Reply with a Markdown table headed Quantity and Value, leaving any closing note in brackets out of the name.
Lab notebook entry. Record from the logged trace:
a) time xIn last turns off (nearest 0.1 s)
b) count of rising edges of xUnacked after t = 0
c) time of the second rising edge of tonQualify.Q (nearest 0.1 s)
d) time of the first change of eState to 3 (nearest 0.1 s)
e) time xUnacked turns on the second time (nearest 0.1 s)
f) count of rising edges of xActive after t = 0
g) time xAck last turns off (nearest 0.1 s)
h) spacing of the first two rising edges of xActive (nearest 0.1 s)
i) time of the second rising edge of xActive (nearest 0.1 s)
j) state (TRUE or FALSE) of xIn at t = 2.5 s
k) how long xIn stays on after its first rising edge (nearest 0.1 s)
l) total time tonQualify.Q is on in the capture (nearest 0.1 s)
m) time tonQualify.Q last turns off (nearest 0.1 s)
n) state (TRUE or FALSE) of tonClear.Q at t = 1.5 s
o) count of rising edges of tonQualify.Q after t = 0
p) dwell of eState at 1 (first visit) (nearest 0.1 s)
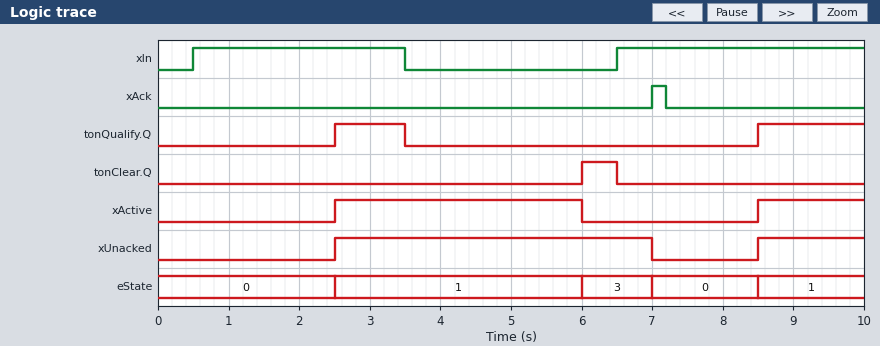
| Quantity | Value |
|---|---|
| time xIn last turns off | 3.5 s |
| count of rising edges of xUnacked after t = 0 | 2 |
| time of the second rising edge of tonQualify.Q | 8.5 s |
| time of the first change of eState to 3 | 6.0 s |
| time xUnacked turns on the second time | 8.5 s |
| count of rising edges of xActive after t = 0 | 2 |
| time xAck last turns off | 7.2 s |
| spacing of the first two rising edges of xActive | 6.0 s |
| time of the second rising edge of xActive | 8.5 s |
| state (TRUE or FALSE) of xIn at t = 2.5 s | TRUE |
| how long xIn stays on after its first rising edge | 3.0 s |
| total time tonQualify.Q is on in the capture | 2.5 s |
| time tonQualify.Q last turns off | 3.5 s |
| state (TRUE or FALSE) of tonClear.Q at t = 1.5 s | FALSE |
| count of rising edges of tonQualify.Q after t = 0 | 2 |
| dwell of eState at 1 (first visit) | 3.5 s |
